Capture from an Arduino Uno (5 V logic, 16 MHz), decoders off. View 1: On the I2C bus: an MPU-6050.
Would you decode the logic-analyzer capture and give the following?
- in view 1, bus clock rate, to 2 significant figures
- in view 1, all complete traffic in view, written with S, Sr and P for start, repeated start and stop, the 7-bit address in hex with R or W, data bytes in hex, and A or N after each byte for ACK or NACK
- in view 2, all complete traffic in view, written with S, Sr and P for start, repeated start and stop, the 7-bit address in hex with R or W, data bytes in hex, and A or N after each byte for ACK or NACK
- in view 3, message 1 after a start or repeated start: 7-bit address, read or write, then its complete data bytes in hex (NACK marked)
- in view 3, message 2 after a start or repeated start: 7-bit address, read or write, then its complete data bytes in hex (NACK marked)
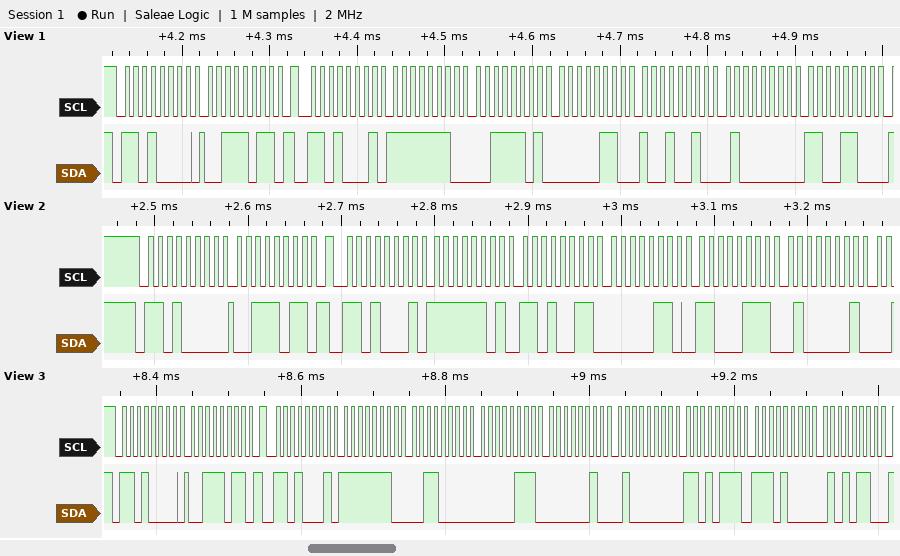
100 kHz
S 68W A 3B A Sr 68R A FE A 3D A 06 A 92 A 40 A CC A
S 68W A 3B A Sr 68R A FD A D3 A 06 A C7 A 41 A
0x68 write: 3B
0x68 read: FE 30 07 02 40 D7 E8 56
